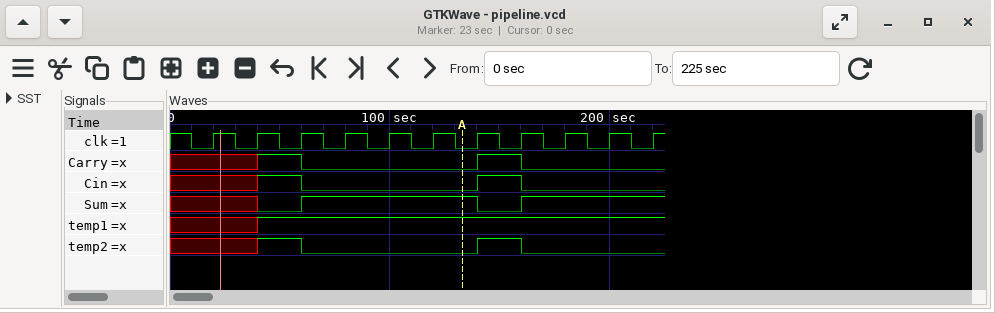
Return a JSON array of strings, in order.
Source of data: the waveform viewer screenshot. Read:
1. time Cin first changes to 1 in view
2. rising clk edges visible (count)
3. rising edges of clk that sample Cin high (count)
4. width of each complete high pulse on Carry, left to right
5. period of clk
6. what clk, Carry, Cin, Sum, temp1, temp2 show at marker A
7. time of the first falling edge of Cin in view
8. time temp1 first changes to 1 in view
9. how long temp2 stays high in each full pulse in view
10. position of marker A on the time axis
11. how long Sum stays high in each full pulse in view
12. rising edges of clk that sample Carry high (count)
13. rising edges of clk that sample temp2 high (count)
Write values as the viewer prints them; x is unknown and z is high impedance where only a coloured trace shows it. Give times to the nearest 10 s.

["40 s", "11", "2", "20 s", "20 s", "clk=0, Carry=0, Cin=0, Sum=1, temp1=1, temp2=0", "60 s", "40 s", "20 s", "130 s", "80 s", "2", "2"]
